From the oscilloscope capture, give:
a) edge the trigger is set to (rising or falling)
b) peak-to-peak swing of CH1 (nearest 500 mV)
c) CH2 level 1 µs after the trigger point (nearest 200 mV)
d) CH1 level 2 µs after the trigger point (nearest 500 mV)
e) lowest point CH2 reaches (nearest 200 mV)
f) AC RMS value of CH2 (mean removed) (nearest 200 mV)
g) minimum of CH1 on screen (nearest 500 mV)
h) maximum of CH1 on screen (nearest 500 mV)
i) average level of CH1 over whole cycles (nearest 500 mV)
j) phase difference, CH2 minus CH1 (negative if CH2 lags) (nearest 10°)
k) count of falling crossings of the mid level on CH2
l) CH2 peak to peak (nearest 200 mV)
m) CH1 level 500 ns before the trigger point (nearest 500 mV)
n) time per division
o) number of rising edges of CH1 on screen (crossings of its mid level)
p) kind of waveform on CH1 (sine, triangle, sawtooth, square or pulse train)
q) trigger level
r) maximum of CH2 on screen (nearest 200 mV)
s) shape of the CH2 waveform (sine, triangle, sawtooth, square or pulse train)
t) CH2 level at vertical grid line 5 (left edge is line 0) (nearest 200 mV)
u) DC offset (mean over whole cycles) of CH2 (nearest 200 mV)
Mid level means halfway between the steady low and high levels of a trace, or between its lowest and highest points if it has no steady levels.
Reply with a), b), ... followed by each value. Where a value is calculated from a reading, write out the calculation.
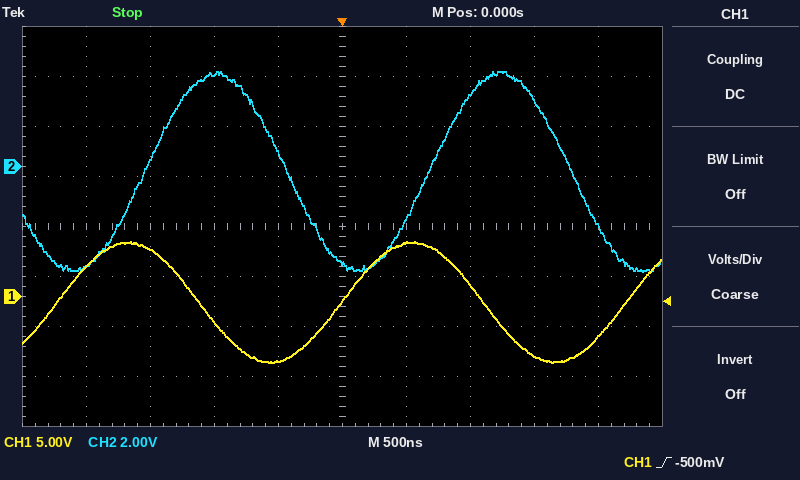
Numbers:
a) rising
b) 5.5 V − (-6.5 V) = 12.0 V
c) 2.8 V
d) -4.0 V
e) -4.2 V
f) 8.0 V / (2√2) ≈ 2.8 V
g) -6.5 V
h) 5.5 V
i) (5.5 V + (-6.5 V)) / 2 ≈ -500 mV
j) -110°
k) 2
l) 3.8 V − (-4.2 V) = 8.0 V
m) -6.5 V
n) 500 ns
o) 3
p) sine
q) -500 mV
r) 3.8 V
s) sine
t) -3.8 V
u) (3.8 V + (-4.2 V)) / 2 ≈ -200 mV
